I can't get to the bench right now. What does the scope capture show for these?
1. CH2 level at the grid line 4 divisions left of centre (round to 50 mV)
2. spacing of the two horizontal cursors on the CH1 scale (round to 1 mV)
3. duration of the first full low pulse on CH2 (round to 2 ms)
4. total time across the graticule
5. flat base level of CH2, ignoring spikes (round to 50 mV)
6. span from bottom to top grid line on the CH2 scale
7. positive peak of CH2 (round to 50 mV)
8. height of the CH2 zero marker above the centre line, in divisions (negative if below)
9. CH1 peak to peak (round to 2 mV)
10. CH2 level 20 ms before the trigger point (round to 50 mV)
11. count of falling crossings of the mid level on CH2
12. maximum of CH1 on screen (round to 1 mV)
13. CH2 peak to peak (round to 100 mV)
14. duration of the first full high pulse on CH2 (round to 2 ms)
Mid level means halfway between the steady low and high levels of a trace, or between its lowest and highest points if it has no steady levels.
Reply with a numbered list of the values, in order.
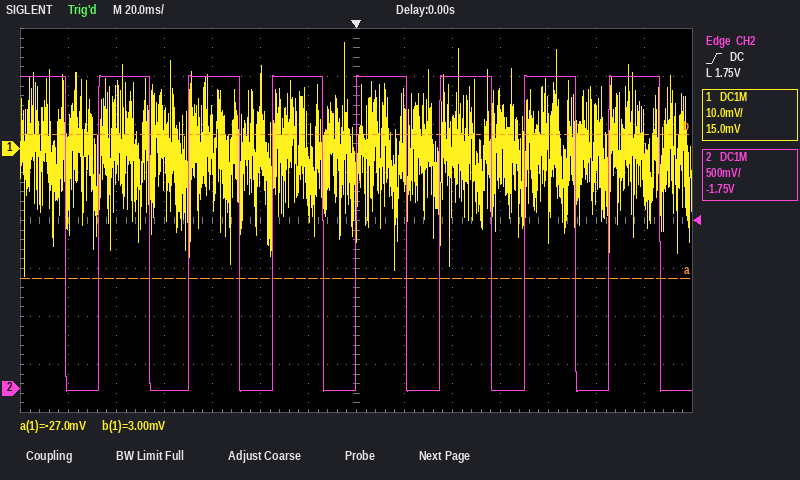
1. 0 mV
2. 30 mV
3. 14 ms
4. 280 ms
5. 0 mV
6. 4 V
7. 3.25 V
8. -3.5 div
9. 48 mV
10. 3.25 V
11. 8
12. 22 mV
13. 3.30 V
14. 22 ms
